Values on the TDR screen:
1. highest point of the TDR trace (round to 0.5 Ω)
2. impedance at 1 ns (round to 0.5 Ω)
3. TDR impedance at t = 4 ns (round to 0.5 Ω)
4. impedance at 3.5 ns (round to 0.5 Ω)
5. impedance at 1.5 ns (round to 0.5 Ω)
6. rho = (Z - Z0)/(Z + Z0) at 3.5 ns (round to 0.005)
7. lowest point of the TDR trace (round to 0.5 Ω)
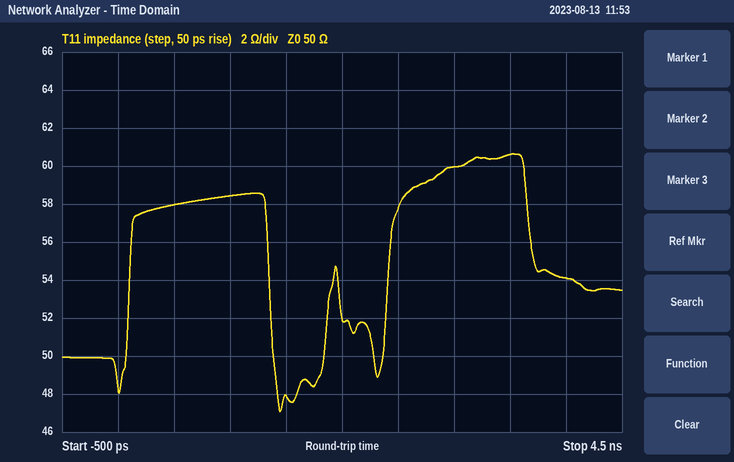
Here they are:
60.5 Ω
58.5 Ω
54.0 Ω
60.5 Ω
48.0 Ω
+0.095
47.0 Ω
